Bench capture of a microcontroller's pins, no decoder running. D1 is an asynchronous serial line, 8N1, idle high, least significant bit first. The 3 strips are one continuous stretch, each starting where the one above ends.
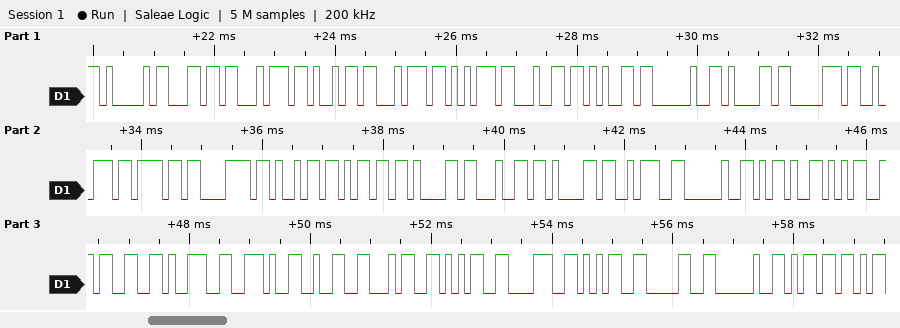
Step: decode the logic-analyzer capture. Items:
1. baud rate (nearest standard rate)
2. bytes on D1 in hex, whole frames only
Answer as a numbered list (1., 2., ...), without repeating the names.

1. 9600 baud
2. 0x41 0x6C 0x74 0x69 0x74 0x75 0x64 0x65 0x20 0x61 0x70 0x72 0x6F 0x78 0x69 0x6D 0x61 0x64 0x61 0x3A 0x20 0x2D 0x35 0x33 0x39 0x2E 0x32 0x34 0x35 0x38 0x35 0x30 0x20 0x6D
